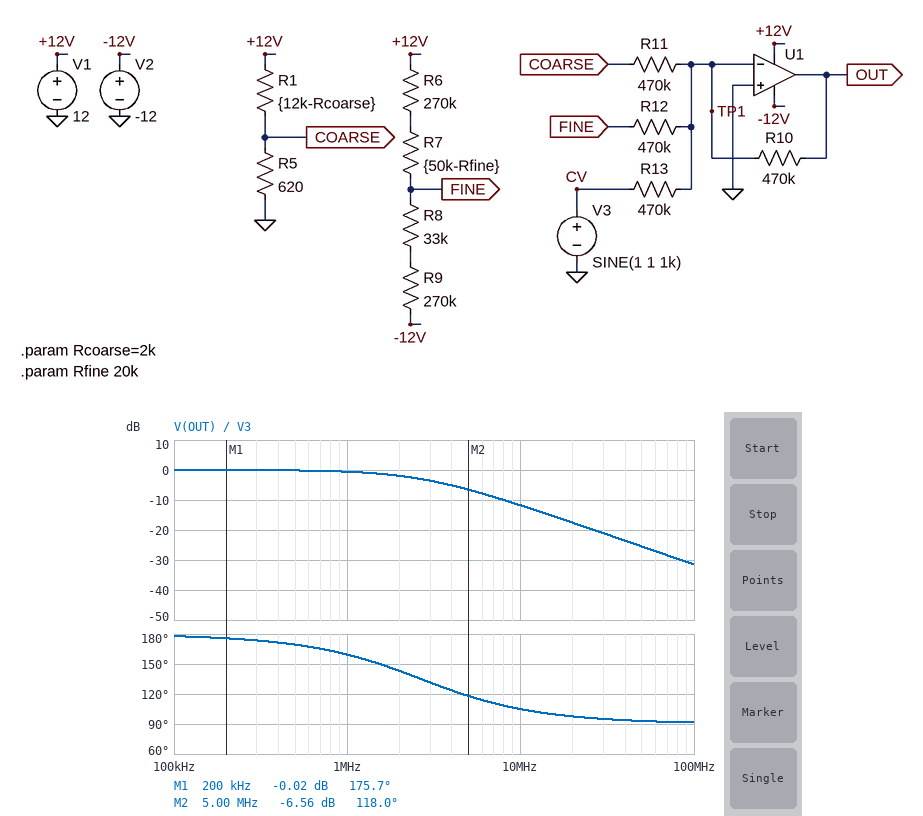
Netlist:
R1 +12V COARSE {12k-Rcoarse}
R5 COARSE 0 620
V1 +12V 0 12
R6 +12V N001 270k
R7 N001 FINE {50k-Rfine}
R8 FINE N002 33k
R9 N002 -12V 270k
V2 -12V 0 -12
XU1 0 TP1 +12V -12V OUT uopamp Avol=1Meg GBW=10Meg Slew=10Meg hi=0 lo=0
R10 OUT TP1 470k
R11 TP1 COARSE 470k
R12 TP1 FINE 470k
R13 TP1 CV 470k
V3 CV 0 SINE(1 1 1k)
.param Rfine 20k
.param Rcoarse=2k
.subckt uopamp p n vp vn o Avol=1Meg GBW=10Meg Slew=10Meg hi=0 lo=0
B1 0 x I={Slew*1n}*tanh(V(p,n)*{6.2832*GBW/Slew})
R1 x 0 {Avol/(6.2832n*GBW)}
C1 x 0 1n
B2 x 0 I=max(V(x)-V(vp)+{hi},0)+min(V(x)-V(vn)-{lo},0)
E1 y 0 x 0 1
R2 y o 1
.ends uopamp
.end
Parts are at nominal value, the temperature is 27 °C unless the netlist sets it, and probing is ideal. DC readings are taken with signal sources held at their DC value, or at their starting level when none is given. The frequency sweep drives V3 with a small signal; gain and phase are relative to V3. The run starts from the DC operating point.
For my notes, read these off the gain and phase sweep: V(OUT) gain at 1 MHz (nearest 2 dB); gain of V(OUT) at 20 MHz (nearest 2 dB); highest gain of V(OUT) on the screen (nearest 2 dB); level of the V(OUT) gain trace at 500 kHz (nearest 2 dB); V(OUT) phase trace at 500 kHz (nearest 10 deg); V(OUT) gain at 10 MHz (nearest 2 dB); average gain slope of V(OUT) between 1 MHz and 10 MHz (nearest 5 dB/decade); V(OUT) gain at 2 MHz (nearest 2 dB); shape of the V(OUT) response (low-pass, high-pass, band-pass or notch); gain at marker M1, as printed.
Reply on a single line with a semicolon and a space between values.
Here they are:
0 dB; -18 dB; 0 dB; 0 dB; 170 deg; -12 dB; -10 dB/decade; -2 dB; low-pass; -0.02 dB
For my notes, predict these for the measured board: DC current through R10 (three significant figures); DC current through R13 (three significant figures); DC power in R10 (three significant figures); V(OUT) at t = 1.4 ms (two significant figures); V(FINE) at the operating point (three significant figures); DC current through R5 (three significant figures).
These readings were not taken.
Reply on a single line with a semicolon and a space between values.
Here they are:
3.71 µA; 2.13 µA; 6.48 µW; -2.3 V; 45.2 mV; 1.13 mA
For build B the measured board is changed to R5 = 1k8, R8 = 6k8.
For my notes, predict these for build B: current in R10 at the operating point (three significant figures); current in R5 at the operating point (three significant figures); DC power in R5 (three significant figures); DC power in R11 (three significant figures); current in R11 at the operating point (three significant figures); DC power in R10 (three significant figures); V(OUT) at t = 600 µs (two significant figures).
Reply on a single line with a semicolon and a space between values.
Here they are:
5.22 µA; 1.01 mA; 1.85 mW; 7.08 µW; 3.88 µA; 12.8 µW; -1.9 V
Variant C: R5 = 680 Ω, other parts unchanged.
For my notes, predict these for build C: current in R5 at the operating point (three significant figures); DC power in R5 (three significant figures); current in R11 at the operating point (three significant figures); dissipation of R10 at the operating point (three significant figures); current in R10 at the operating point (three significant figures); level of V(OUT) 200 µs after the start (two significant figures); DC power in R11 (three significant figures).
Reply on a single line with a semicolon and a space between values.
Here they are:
1.12 mA; 856 µW; 1.62 µA; 6.96 µW; 3.85 µA; -2.8 V; 1.24 µW
